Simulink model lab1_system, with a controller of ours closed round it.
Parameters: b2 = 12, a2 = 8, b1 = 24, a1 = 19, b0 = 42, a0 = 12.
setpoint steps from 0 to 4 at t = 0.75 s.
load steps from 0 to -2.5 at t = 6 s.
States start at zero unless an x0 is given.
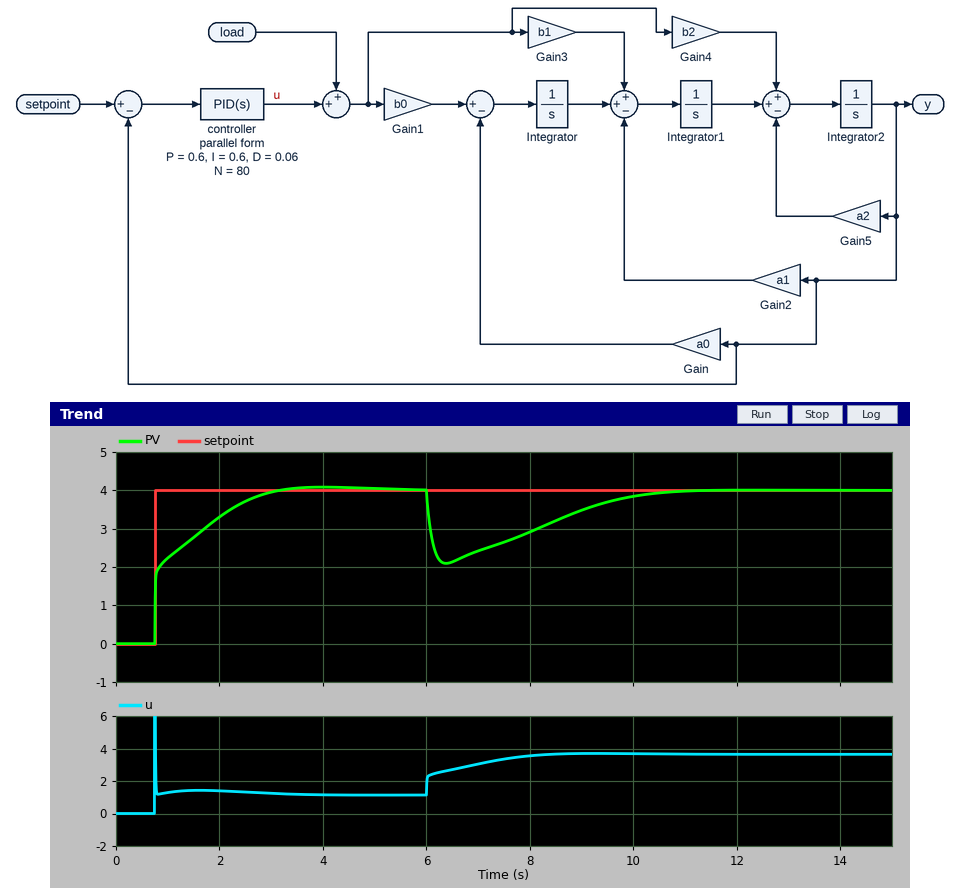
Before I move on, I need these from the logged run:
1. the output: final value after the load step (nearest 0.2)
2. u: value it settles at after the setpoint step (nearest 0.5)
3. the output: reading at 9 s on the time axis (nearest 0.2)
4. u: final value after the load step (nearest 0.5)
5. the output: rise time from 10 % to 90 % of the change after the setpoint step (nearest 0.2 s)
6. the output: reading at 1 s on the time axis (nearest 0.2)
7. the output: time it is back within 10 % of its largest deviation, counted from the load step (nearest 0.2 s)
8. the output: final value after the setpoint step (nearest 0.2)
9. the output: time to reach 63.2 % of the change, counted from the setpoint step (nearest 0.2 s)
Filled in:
4.0
1.0
3.4
3.5
1.6 s
2.2
3.8 s
4.0
0.6 s
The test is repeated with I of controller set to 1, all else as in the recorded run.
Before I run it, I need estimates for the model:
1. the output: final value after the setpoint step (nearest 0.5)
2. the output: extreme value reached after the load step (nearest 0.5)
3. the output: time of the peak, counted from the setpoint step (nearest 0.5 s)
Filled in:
4.0
2.0
2.5 s
